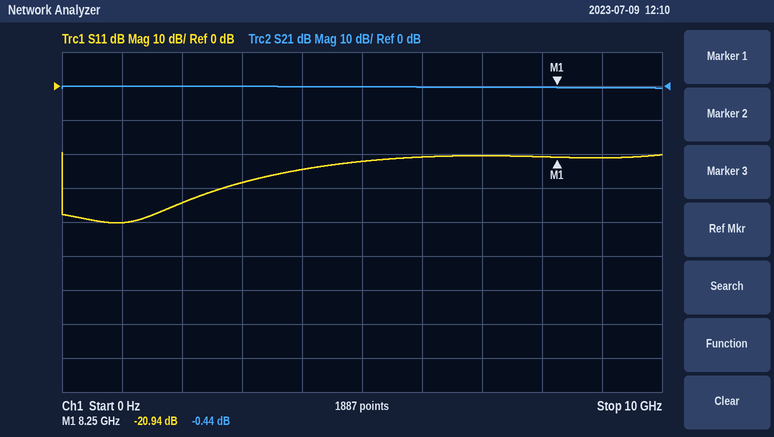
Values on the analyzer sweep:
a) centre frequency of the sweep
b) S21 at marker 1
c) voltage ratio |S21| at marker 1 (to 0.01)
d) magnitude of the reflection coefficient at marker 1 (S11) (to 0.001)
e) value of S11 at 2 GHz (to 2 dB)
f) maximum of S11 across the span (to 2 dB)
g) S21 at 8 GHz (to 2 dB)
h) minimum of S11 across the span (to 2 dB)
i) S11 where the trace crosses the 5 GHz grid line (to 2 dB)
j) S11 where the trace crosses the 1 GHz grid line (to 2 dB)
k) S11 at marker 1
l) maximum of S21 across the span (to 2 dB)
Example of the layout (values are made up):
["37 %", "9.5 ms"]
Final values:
["5 GHz", "-0.44 dB", "0.95", "0.090", "-34 dB", "-20 dB", "0 dB", "-40 dB", "-22 dB", "-40 dB", "-20.94 dB", "0 dB"]
